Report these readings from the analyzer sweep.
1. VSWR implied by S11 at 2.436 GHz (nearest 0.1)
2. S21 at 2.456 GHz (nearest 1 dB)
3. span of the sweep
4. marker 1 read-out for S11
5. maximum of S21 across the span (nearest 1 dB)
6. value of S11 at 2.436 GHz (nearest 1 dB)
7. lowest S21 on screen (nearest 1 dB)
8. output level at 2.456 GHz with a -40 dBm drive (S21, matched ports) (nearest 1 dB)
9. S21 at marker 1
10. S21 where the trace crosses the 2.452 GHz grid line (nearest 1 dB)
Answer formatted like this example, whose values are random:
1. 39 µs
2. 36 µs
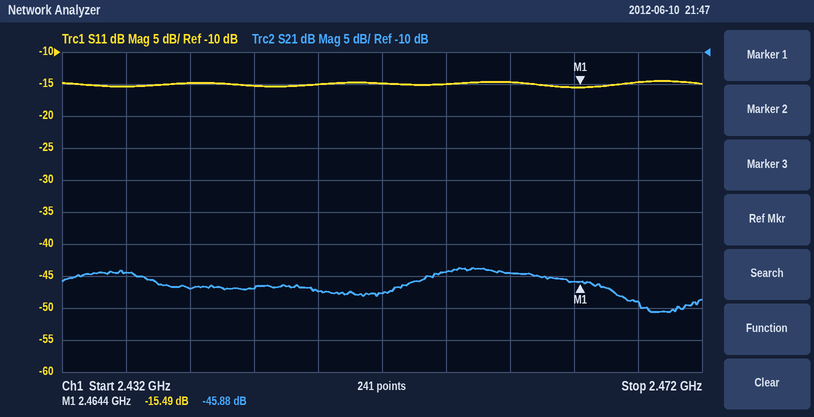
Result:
1. 1.4
2. -44 dB
3. 40 MHz
4. -15.49 dB
5. -44 dB
6. -15 dB
7. -51 dB
8. -84 dBm
9. -45.88 dB
10. -48 dB
